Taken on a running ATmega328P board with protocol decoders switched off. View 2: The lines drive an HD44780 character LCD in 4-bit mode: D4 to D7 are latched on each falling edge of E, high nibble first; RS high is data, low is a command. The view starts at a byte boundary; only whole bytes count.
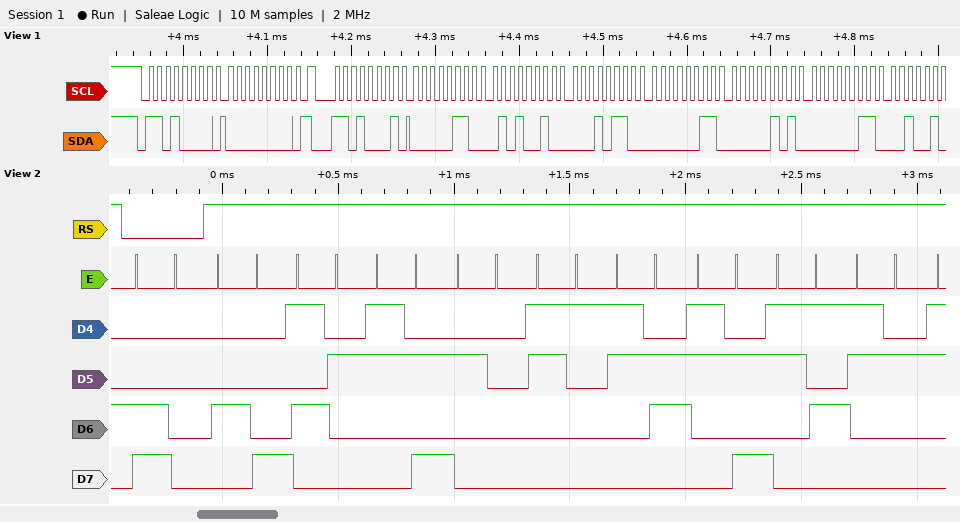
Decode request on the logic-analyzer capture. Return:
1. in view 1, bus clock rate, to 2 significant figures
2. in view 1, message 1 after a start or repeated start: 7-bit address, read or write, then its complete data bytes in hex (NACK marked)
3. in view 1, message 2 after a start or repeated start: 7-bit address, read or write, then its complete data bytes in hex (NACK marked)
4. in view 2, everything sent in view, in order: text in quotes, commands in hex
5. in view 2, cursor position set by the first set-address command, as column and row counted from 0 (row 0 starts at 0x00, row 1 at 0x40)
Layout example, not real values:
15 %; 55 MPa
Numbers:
100 kHz; 0x68 write: 00; 0x68 read: 06 52 16 03 05 03; 0xC0 "HR: 16:52"; column 0, row 1
